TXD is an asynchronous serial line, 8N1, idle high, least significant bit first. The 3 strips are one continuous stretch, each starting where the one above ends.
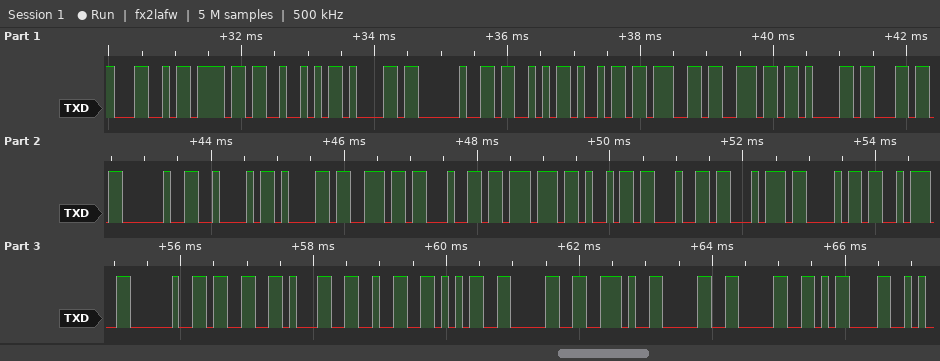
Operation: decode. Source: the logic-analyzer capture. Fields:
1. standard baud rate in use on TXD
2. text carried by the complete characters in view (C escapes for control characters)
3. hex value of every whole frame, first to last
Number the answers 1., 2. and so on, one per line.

1. 9600 baud
2. "LoRa Signal Bandwidth: 31250.00\r"
3. 4C 6F 52 61 20 53 69 67 6E 61 6C 20 42 61 6E 64 77 69 64 74 68 3A 20 33 31 32 35 30 2E 30 30 0D
